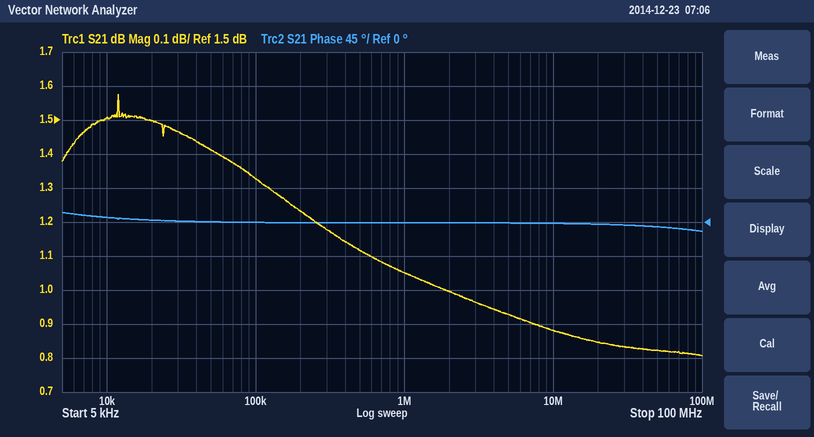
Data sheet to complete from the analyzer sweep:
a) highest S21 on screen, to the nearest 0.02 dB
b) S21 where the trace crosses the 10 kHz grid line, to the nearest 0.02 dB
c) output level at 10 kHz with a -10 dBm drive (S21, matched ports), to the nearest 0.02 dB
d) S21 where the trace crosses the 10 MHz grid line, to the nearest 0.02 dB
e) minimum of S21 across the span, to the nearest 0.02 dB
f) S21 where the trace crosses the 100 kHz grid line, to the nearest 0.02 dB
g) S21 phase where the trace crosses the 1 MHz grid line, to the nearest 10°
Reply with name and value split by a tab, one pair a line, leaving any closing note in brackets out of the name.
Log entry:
highest S21 on screen, to the nearest 0.02 dB	1.58 dB
S21 where the trace crosses the 10 kHz grid line, to the nearest 0.02 dB	1.50 dB
output level at 10 kHz with a -10 dBm drive (S21, matched ports), to the nearest 0.02 dB	-8.50 dBm
S21 where the trace crosses the 10 MHz grid line, to the nearest 0.02 dB	0.88 dB
minimum of S21 across the span, to the nearest 0.02 dB	0.80 dB
S21 where the trace crosses the 100 kHz grid line, to the nearest 0.02 dB	1.32 dB
S21 phase where the trace crosses the 1 MHz grid line, to the nearest 10°	0°
